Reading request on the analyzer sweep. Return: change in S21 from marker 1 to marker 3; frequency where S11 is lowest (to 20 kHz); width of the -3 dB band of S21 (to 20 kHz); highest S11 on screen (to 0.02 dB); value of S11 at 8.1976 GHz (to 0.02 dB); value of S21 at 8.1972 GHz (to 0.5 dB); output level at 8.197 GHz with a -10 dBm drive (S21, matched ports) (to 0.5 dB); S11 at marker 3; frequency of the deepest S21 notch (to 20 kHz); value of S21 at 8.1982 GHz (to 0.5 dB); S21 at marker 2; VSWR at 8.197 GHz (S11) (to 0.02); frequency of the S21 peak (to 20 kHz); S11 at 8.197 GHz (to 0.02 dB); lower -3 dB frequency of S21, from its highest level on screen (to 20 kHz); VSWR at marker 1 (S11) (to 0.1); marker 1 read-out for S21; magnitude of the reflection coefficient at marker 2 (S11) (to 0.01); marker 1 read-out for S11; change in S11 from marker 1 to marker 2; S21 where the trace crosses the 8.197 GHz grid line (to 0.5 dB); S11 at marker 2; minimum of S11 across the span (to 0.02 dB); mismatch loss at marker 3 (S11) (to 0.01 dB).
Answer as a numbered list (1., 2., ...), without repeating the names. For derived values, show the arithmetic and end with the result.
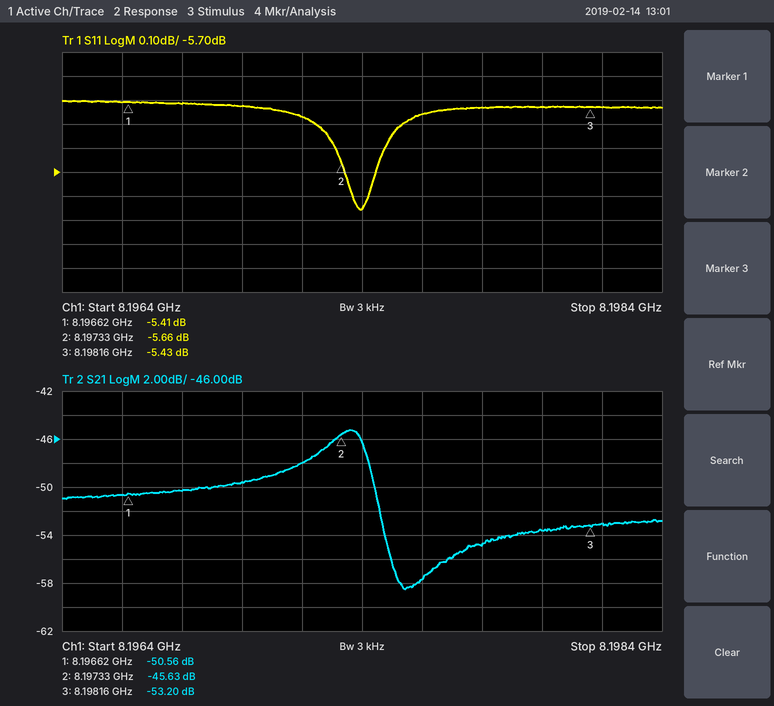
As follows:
1. -53.2 − (-50.56) = -2.64 dB
2. 8.19740 GHz
3. 8.19742 GHz − 8.19718 GHz = 240 kHz
4. -5.40 dB
5. -5.46 dB
6. -48.0 dB
7. -10 dBm + (-49.5 dB) = -59.5 dBm
8. -5.43 dB
9. 8.19754 GHz
10. -53.0 dB
11. -45.63 dB
12. |Γ| = 10^(-5.42/20) = 0.5358; VSWR = (1 + 0.5358)/(1 − 0.5358) ≈ 3.31, so 3.30 to the nearest 0.02
13. 8.19736 GHz
14. -5.42 dB
15. 8.19718 GHz
16. (1 + 0.5364)/(1 − 0.5364) ≈ 3.3
17. -50.56 dB
18. 10^(-5.66/20) ≈ 0.52
19. -5.41 dB
20. -5.66 − (-5.41) = -0.25 dB
21. -49.5 dB
22. -5.66 dB
23. -5.86 dB
24. −10 log10(1 − 10^(-5.43/10)) ≈ 1.47 dB
